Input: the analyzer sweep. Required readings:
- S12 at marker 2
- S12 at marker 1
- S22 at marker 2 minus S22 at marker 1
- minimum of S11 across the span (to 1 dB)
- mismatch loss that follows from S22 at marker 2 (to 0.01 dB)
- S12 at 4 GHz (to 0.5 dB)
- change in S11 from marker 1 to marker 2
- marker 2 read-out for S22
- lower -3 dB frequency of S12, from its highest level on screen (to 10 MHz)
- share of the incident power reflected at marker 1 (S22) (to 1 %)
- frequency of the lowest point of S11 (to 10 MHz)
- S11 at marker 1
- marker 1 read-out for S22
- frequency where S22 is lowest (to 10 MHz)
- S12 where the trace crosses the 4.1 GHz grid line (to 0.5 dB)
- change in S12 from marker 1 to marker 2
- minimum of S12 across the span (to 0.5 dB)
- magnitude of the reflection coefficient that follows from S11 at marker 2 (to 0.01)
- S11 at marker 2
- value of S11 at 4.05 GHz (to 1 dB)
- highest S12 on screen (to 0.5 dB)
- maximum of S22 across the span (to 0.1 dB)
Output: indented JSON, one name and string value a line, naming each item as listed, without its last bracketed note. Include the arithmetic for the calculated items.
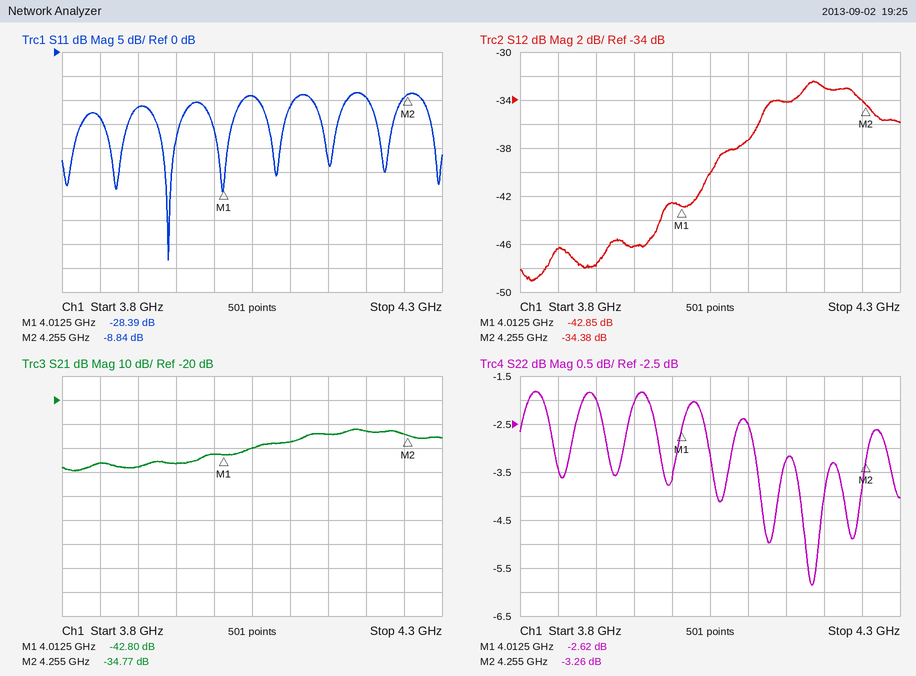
{
  "S12 at marker 2": "-34.38 dB",
  "S12 at marker 1": "-42.85 dB",
  "S22 at marker 2 minus S22 at marker 1": "-3.26 − (-2.62) = -0.64 dB",
  "minimum of S11 across the span": "-43 dB",
  "mismatch loss that follows from S22 at marker 2": "−10 log10(1 − 10^(-3.26/10)) ≈ 2.77 dB",
  "S12 at 4 GHz": "-42.5 dB",
  "change in S11 from marker 1 to marker 2": "-8.84 − (-28.39) = 19.55 dB",
  "marker 2 read-out for S22": "-3.26 dB",
  "lower -3 dB frequency of S12, from its highest level on screen": "4.12 GHz",
  "share of the incident power reflected at marker 1 (S22)": "10^(-2.62/10) ≈ 55 %",
  "frequency of the lowest point of S11": "3.94 GHz",
  "S11 at marker 1": "-28.39 dB",
  "marker 1 read-out for S22": "-2.62 dB",
  "frequency where S22 is lowest": "4.18 GHz",
  "S12 where the trace crosses the 4.1 GHz grid line": "-37.5 dB",
  "change in S12 from marker 1 to marker 2": "-34.38 − (-42.85) = 8.47 dB",
  "minimum of S12 across the span": "-49.0 dB",
  "magnitude of the reflection coefficient that follows from S11 at marker 2": "10^(-8.84/20) ≈ 0.36",
  "S11 at marker 2": "-8.84 dB",
  "value of S11 at 4.05 GHz": "-9 dB",
  "highest S12 on screen": "-32.5 dB",
  "maximum of S22 across the span": "-1.8 dB"
}
